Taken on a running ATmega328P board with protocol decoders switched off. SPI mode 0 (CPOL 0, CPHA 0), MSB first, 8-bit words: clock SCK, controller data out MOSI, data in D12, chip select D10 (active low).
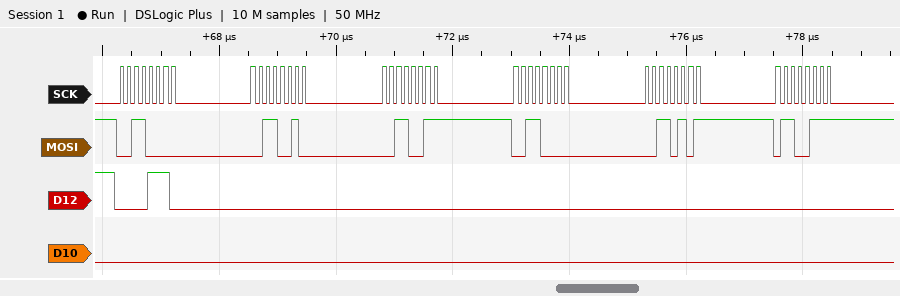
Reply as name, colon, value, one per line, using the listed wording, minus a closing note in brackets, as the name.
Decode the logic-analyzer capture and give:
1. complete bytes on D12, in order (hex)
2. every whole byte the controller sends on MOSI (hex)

complete bytes on D12, in order: 0x0E 0x00 0x00 0x00 0x00 0x00
every whole byte the controller sends on MOSI: 0x30 0x32 0x33 0x30 0x35 0x67
